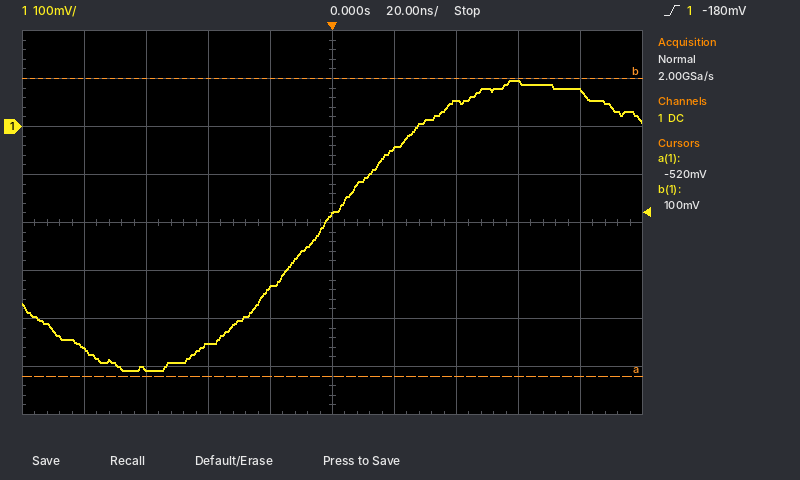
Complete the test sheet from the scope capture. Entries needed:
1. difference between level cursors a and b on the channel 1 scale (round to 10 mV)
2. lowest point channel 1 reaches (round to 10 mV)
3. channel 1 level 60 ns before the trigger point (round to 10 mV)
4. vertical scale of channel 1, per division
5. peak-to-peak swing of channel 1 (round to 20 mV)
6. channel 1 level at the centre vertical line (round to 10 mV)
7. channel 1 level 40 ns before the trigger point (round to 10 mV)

620 mV
-510 mV
-500 mV
100 mV
600 mV
-180 mV
-450 mV
